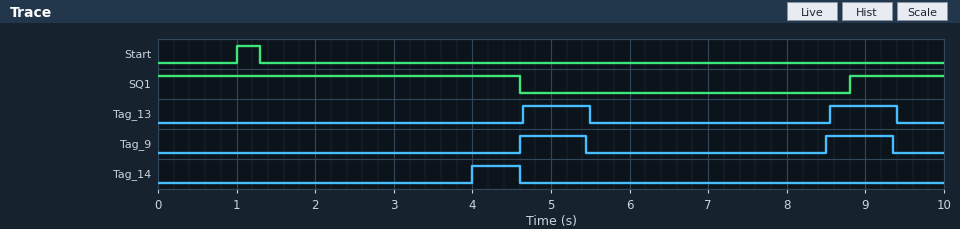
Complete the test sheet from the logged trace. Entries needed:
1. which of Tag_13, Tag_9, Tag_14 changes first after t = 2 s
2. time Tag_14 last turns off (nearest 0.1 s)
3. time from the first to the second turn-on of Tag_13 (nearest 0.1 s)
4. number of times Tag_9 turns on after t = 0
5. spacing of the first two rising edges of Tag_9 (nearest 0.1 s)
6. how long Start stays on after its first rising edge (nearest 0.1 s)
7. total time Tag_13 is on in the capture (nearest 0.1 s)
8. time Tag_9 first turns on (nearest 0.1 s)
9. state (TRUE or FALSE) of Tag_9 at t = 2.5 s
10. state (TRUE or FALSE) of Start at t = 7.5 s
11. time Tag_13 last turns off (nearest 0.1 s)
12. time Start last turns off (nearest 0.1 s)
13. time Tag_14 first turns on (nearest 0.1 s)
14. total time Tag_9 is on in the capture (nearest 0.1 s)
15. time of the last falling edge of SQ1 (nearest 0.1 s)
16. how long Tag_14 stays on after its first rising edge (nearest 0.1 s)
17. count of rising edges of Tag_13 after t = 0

Tag_14
4.6 s
3.9 s
2
3.9 s
0.3 s
1.7 s
4.6 s
FALSE
FALSE
9.4 s
1.3 s
4.0 s
1.7 s
4.6 s
0.6 s
2
